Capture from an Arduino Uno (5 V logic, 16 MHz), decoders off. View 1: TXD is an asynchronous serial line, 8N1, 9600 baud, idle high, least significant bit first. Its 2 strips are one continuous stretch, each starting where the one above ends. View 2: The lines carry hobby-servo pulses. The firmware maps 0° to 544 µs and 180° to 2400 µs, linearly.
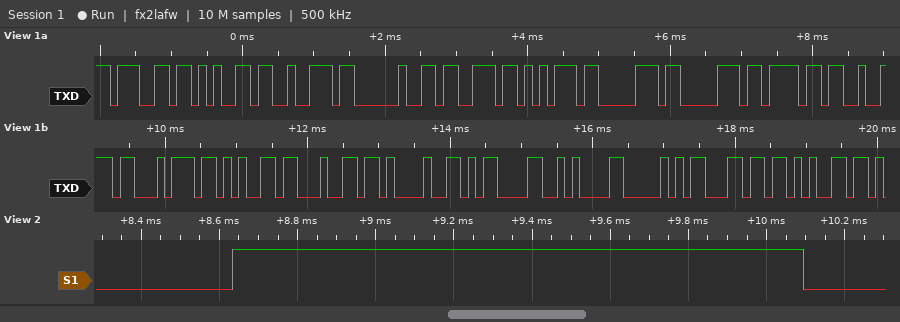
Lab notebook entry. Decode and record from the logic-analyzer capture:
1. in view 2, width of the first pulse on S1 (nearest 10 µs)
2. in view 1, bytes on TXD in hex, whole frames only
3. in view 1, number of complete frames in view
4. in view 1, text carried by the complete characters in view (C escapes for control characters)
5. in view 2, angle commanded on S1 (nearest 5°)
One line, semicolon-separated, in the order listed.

1460 µs; 0x67 0x65 0x72 0x20 0x73 0x75 0x70 0x70 0x6F 0x72 0x74 0x65 0x64 0x21 0x0D 0x0A 0x50 0x6C 0x65; 19; "ger supported!\r\nPle"; 90°
